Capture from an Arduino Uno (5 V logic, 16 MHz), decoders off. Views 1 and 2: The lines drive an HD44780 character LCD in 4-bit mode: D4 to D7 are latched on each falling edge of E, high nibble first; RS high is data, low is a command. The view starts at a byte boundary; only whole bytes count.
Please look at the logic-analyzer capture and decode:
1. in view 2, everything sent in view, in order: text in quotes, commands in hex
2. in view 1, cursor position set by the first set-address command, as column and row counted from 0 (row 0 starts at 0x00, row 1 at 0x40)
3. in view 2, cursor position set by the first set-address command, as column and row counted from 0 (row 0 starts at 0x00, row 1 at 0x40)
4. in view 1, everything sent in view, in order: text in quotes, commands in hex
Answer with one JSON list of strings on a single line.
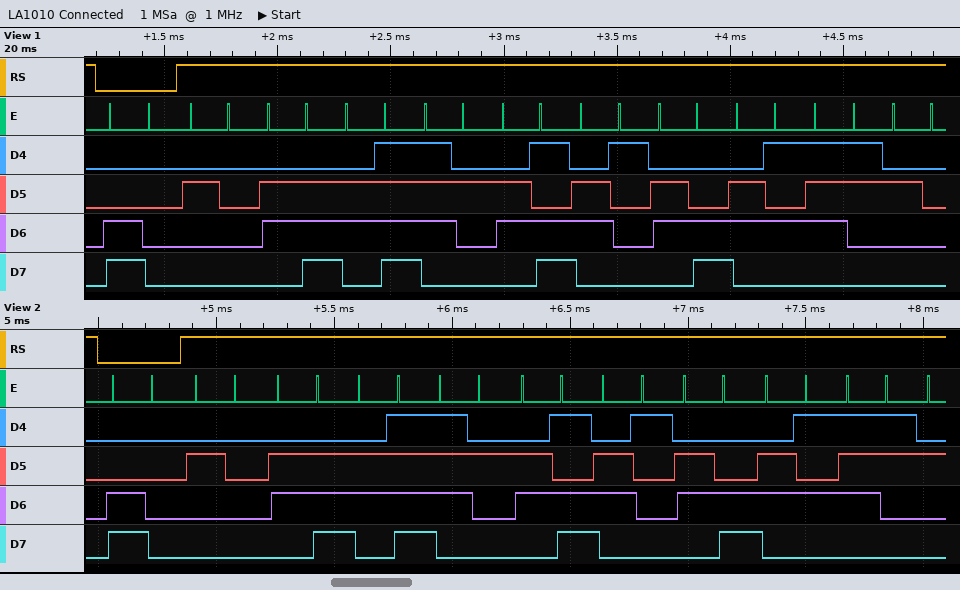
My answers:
["0xC0 \" normales\"", "column 0, row 1", "column 0, row 1", "0xC0 \" normales \""]
